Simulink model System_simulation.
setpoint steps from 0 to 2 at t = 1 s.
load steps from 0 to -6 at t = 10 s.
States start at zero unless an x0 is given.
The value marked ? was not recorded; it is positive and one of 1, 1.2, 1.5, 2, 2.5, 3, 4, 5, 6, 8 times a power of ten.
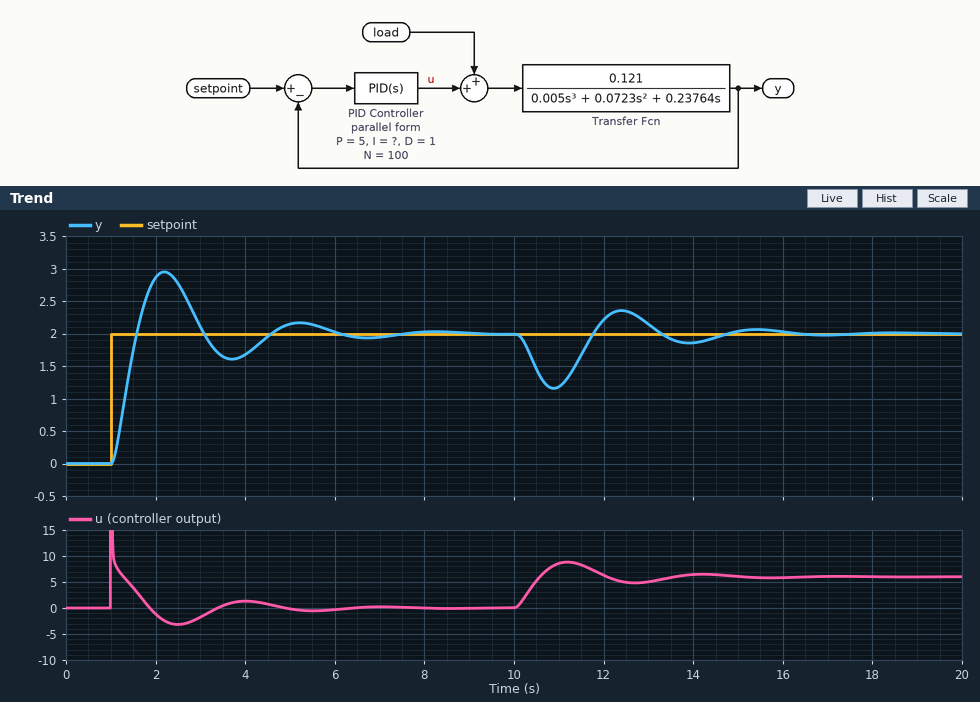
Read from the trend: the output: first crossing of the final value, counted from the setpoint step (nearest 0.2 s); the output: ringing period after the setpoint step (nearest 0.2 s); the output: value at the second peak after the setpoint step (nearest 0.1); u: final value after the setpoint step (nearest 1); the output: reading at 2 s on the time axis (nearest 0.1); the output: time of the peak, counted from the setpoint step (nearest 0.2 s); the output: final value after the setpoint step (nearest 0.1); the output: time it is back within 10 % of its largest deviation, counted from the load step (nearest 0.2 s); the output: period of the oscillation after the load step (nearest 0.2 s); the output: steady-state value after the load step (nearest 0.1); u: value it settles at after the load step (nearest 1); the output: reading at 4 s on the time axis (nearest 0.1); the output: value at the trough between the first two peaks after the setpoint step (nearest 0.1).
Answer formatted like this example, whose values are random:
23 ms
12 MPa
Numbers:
0.6 s
3.0 s
2.2
0
2.9
1.2 s
2.0
4.4 s
3.0 s
2.0
6
1.7
1.6
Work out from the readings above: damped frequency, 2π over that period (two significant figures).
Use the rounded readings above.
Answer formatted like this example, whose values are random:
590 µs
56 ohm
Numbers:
2.1 rad/s
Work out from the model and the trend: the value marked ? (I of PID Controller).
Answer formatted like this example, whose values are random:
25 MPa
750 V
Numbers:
10
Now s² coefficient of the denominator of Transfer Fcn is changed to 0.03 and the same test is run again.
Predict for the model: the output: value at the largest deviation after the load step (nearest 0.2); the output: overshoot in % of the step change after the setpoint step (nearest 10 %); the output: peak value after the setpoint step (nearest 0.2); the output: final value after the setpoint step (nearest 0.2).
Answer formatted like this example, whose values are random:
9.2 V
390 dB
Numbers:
1.2
30 %
2.6
2.0
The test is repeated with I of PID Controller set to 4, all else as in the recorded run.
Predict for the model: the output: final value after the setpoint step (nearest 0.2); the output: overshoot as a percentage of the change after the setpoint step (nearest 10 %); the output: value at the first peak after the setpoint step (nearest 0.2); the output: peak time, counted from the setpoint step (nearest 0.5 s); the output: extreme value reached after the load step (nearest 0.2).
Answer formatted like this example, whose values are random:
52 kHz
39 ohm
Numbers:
2.0
20 %
2.4
1.5 s
1.0
